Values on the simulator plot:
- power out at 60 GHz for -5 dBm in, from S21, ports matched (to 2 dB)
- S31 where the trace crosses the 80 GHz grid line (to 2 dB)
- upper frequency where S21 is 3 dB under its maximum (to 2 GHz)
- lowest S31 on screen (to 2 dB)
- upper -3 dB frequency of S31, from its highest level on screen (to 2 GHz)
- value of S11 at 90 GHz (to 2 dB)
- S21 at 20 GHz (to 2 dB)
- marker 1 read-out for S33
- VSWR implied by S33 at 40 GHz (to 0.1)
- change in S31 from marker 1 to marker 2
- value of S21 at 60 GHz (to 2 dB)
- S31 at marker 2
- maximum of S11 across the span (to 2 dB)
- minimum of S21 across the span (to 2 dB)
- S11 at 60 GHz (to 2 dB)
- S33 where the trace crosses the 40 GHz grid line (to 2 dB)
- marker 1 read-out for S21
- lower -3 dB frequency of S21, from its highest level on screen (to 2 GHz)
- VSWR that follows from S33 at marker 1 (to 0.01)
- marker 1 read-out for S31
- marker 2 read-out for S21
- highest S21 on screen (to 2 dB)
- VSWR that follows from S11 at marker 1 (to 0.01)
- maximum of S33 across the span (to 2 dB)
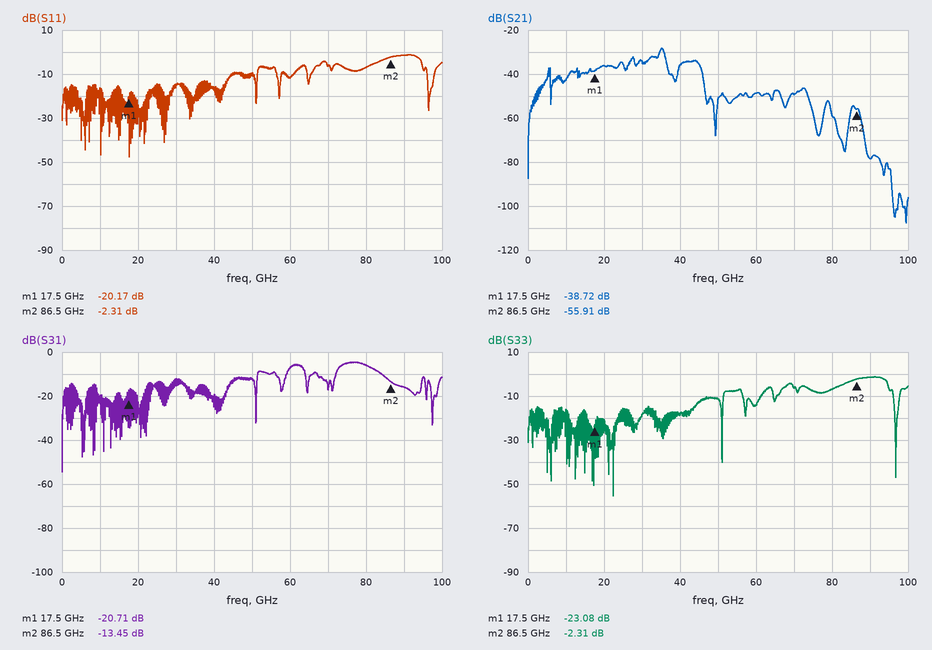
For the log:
-54 dBm
-6 dB
36 GHz
-54 dB
82 GHz
-2 dB
-36 dB
-23.08 dB
1.3
7.26 dB
-48 dB
-13.45 dB
-2 dB
-108 dB
-12 dB
-18 dB
-38.72 dB
34 GHz
1.15
-20.71 dB
-55.91 dB
-28 dB
1.22
-2 dB
